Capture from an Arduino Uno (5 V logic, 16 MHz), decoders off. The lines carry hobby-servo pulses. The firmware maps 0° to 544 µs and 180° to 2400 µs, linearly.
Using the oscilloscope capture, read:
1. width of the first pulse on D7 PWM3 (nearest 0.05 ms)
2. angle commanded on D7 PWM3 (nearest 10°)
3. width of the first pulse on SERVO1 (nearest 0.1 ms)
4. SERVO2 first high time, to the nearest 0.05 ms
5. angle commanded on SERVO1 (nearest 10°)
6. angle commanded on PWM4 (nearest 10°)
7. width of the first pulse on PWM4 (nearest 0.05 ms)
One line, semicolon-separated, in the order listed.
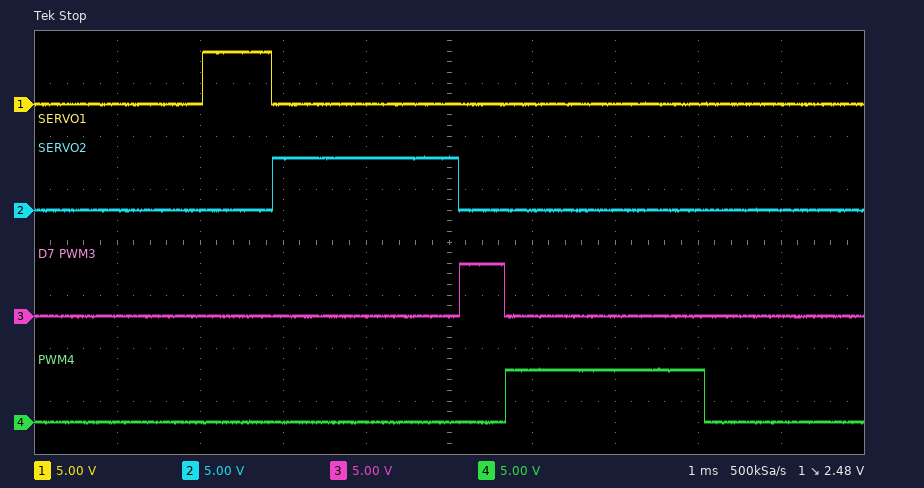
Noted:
0.55 ms; 0°; 0.8 ms; 2.25 ms; 30°; 180°; 2.40 ms
